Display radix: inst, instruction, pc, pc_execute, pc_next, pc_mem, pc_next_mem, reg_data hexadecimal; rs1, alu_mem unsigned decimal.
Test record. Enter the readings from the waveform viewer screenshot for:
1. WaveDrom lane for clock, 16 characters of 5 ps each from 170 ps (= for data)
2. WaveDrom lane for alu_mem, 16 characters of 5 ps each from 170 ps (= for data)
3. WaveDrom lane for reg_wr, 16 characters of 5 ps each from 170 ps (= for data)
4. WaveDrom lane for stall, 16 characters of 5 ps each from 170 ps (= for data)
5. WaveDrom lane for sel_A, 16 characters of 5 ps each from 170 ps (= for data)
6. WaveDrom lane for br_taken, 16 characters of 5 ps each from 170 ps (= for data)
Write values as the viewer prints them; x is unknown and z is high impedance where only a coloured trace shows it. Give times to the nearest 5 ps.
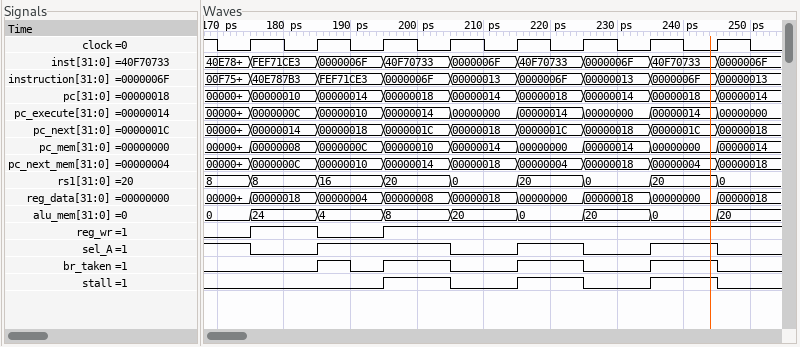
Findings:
{name: 'clock', wave: '0101010101010101'}
{name: 'alu_mem', wave: '==.=.=.=.=.=.=.=', data: '0 24 4 8 20 0 20 0 20'}
{name: 'reg_wr', wave: '01.0.1..........'}
{name: 'stall', wave: '0....1.0.1.0.1.0'}
{name: 'sel_A', wave: '10.1...0.1.0.1.0'}
{name: 'br_taken', wave: '0..101.0.1.0.1.0'}
